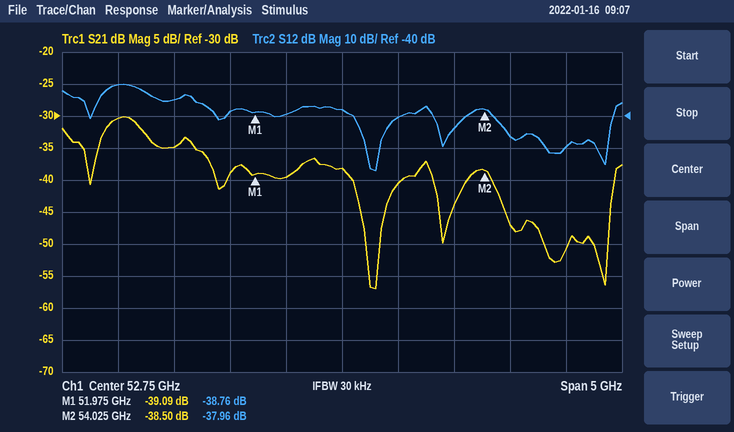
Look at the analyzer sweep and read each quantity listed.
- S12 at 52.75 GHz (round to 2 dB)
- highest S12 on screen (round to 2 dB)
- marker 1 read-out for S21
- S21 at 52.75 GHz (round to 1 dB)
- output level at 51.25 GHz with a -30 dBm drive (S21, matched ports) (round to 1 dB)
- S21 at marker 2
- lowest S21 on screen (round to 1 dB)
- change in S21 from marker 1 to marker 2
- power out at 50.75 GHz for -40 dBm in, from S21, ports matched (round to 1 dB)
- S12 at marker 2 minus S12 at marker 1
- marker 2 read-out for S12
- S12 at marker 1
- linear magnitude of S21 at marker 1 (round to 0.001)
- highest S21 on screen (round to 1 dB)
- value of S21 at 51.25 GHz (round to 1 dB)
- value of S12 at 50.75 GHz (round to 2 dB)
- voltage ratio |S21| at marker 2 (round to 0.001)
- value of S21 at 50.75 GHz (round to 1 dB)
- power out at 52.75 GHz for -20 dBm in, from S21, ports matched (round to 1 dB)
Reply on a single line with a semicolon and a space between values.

-38 dB; -30 dB; -39.09 dB; -38 dB; -65 dBm; -38.50 dB; -57 dB; 0.59 dB; -70 dBm; 0.80 dB; -37.96 dB; -38.76 dB; 0.011; -30 dB; -35 dB; -30 dB; 0.012; -30 dB; -58 dBm
